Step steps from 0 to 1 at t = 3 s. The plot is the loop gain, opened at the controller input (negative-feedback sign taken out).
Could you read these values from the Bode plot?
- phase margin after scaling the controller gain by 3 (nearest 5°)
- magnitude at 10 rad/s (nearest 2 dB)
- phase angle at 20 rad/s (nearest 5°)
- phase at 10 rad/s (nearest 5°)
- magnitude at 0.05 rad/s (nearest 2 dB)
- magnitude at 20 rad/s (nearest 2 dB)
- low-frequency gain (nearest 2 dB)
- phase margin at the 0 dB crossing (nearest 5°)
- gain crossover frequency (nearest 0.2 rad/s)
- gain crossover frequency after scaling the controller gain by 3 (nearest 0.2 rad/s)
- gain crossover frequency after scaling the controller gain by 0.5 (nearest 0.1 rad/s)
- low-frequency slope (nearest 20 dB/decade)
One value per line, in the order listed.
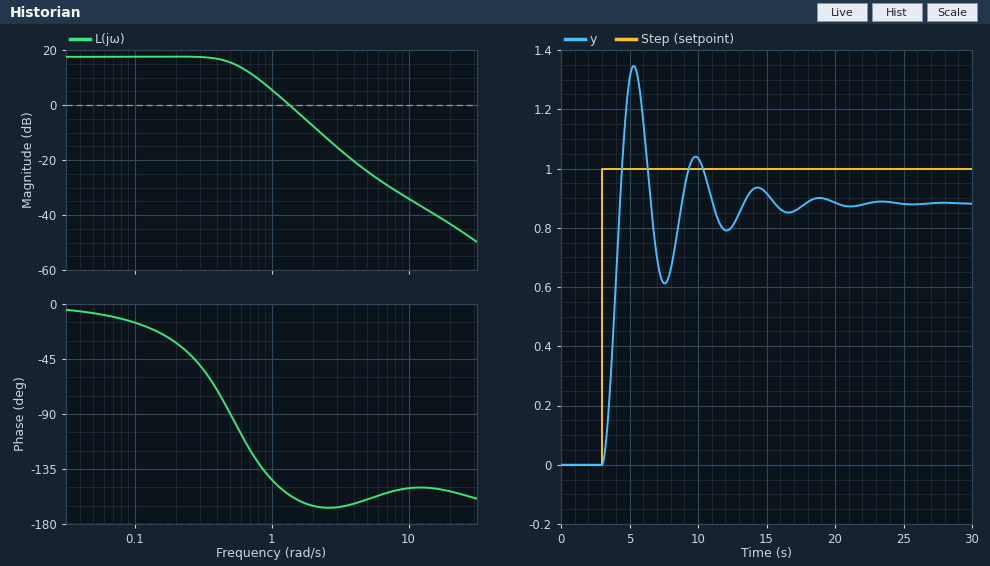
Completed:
15°
-34 dB
-155°
-150°
18 dB
-44 dB
18 dB
25°
1.4 rad/s
2.2 rad/s
1.0 rad/s
0 dB/decade
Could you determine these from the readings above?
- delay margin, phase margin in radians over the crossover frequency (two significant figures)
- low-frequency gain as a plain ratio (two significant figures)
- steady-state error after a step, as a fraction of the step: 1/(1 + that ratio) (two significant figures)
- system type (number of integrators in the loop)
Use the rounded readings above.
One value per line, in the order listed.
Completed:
0.31 s
7.9
0.11
0
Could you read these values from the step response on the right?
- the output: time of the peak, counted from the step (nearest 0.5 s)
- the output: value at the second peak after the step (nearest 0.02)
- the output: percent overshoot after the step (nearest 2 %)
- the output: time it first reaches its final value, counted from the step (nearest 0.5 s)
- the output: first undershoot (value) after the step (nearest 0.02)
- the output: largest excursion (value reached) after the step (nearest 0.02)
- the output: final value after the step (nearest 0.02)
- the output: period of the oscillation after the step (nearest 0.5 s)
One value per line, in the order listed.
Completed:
2.5 s
1.04
52 %
1.5 s
0.62
1.34
0.88
4.5 s
